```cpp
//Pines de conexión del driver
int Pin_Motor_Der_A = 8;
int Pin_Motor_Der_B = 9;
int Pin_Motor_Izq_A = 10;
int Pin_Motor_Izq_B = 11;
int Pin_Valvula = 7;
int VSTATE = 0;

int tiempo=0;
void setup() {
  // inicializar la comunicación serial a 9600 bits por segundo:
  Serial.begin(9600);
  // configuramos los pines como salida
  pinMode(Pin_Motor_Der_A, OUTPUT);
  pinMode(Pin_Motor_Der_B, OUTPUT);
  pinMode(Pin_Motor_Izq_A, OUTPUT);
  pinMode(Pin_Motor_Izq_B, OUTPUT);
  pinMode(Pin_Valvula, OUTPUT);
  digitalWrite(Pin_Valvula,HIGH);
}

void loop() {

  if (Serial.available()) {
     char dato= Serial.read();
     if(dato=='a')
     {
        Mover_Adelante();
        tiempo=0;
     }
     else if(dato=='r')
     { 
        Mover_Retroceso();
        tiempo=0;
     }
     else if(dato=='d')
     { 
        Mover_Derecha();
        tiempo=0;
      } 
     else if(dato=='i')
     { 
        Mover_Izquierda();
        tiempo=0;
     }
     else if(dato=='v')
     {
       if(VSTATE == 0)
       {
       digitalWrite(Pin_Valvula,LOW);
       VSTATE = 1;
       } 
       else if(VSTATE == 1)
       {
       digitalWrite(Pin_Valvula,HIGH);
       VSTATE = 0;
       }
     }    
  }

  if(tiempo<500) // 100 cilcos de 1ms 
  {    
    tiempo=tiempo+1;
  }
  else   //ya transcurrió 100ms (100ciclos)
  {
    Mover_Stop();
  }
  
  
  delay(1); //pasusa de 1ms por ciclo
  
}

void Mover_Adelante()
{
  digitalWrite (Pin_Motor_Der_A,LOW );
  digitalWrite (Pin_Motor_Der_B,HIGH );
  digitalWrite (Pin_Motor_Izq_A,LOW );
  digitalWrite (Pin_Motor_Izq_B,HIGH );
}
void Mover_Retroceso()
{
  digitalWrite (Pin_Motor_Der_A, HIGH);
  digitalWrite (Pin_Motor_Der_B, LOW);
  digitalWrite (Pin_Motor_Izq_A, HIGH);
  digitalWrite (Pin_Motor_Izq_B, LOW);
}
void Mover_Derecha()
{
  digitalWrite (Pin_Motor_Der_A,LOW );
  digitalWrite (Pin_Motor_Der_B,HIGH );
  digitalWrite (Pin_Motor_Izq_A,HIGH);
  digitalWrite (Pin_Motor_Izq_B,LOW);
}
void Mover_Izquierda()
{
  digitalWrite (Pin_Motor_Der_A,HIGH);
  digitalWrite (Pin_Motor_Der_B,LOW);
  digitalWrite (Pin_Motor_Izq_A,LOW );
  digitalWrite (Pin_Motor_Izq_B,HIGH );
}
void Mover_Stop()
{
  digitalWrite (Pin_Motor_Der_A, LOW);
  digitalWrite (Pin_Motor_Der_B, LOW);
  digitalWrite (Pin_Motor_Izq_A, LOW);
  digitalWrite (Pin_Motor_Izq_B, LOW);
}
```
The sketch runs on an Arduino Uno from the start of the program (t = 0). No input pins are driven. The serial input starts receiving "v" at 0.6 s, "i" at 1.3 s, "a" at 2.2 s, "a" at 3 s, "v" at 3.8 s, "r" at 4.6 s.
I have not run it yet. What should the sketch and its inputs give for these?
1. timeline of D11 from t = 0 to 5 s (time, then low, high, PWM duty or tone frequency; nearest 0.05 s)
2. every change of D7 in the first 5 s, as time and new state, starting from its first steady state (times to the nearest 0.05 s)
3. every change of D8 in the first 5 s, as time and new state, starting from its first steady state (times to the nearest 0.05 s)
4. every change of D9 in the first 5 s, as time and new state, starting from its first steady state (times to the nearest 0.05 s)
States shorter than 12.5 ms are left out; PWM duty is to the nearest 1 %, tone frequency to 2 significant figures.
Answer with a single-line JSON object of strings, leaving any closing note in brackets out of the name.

{"timeline of D11 from t = 0 to 5 s": "0 s low; 1.3 s high; 1.8 s low; 2.2 s high; 2.7 s low; 3 s high; 3.5 s low", "every change of D7 in the first 5 s, as time and new state, starting from its first steady state": "0 s high; 0.6 s low; 3.8 s high", "every change of D8 in the first 5 s, as time and new state, starting from its first steady state": "0 s low; 1.3 s high; 1.8 s low; 4.6 s high", "every change of D9 in the first 5 s, as time and new state, starting from its first steady state": "0 s low; 2.2 s high; 2.7 s low; 3 s high; 3.5 s low"}
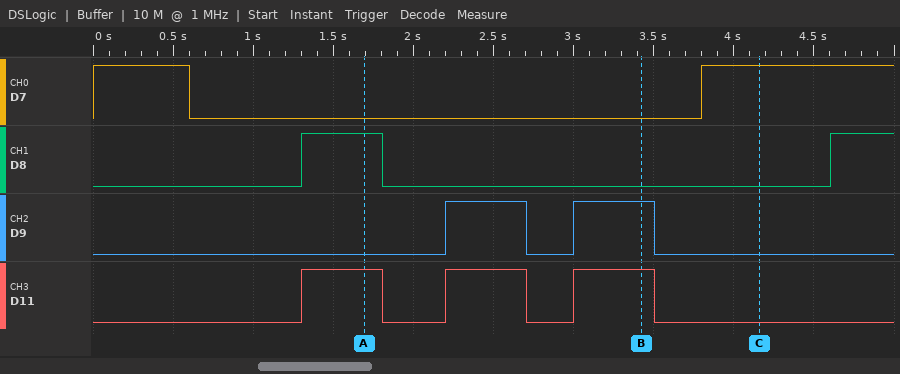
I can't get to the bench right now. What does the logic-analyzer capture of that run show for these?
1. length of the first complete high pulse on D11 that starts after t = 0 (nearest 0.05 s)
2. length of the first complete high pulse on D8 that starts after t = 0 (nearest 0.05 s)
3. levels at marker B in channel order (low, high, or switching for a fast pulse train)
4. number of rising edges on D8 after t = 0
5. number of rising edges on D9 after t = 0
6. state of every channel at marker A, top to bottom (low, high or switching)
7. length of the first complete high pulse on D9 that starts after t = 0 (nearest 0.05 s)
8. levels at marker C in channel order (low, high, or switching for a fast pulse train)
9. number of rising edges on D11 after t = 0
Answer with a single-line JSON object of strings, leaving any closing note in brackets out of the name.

{"length of the first complete high pulse on D11 that starts after t = 0": "0.50 s", "length of the first complete high pulse on D8 that starts after t = 0": "0.50 s", "levels at marker B in channel order": "D7 low, D8 low, D9 high, D11 high", "number of rising edges on D8 after t = 0": "2", "number of rising edges on D9 after t = 0": "2", "state of every channel at marker A, top to bottom": "D7 low, D8 high, D9 low, D11 high", "length of the first complete high pulse on D9 that starts after t = 0": "0.50 s", "levels at marker C in channel order": "D7 high, D8 low, D9 low, D11 low", "number of rising edges on D11 after t = 0": "3"}
